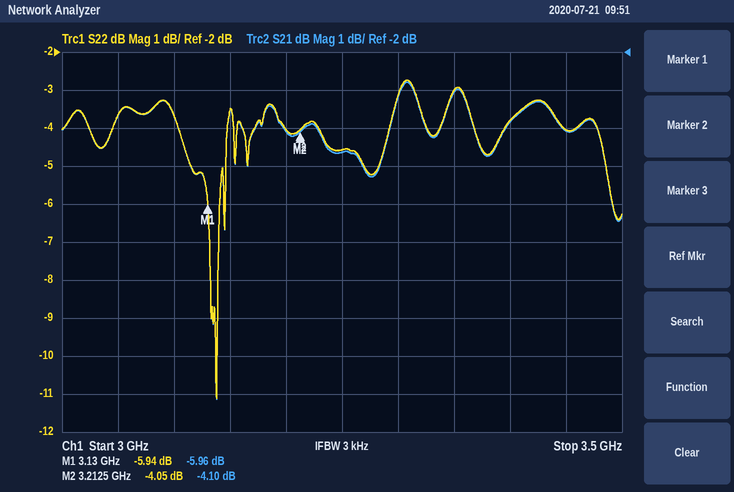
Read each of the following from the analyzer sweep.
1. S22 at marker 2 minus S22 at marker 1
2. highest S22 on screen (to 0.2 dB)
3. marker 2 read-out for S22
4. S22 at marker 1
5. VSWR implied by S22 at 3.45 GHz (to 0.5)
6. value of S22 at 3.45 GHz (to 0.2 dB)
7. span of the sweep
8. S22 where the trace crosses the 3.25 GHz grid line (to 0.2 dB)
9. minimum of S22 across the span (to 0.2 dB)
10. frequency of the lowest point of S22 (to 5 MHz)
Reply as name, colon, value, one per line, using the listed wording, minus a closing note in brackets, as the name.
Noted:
S22 at marker 2 minus S22 at marker 1: 1.89 dB
highest S22 on screen: -2.8 dB
marker 2 read-out for S22: -4.05 dB
S22 at marker 1: -5.94 dB
VSWR implied by S22 at 3.45 GHz: 4.5
value of S22 at 3.45 GHz: -4.0 dB
span of the sweep: 500 MHz
S22 where the trace crosses the 3.25 GHz grid line: -4.6 dB
minimum of S22 across the span: -11.2 dB
frequency of the lowest point of S22: 3.140 GHz
